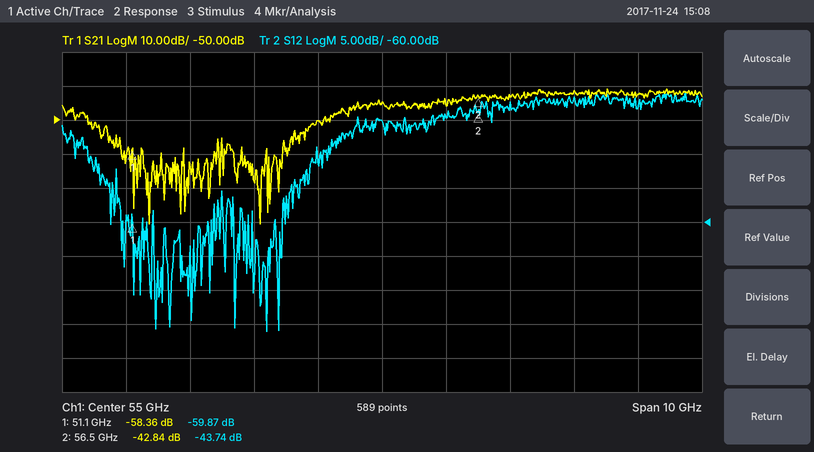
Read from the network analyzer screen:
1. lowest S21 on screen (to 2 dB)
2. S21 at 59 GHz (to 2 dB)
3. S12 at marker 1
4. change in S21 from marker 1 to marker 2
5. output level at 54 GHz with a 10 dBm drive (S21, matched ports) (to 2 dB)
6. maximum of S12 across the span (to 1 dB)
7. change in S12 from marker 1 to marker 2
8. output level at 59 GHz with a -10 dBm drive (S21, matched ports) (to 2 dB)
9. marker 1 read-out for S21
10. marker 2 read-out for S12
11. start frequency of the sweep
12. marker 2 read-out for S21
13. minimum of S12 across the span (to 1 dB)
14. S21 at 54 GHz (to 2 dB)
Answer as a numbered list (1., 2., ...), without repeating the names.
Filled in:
1. -80 dB
2. -42 dB
3. -59.87 dB
4. 15.52 dB
5. -40 dBm
6. -41 dB
7. 16.13 dB
8. -52 dBm
9. -58.36 dB
10. -43.74 dB
11. 50 GHz
12. -42.84 dB
13. -76 dB
14. -50 dB
